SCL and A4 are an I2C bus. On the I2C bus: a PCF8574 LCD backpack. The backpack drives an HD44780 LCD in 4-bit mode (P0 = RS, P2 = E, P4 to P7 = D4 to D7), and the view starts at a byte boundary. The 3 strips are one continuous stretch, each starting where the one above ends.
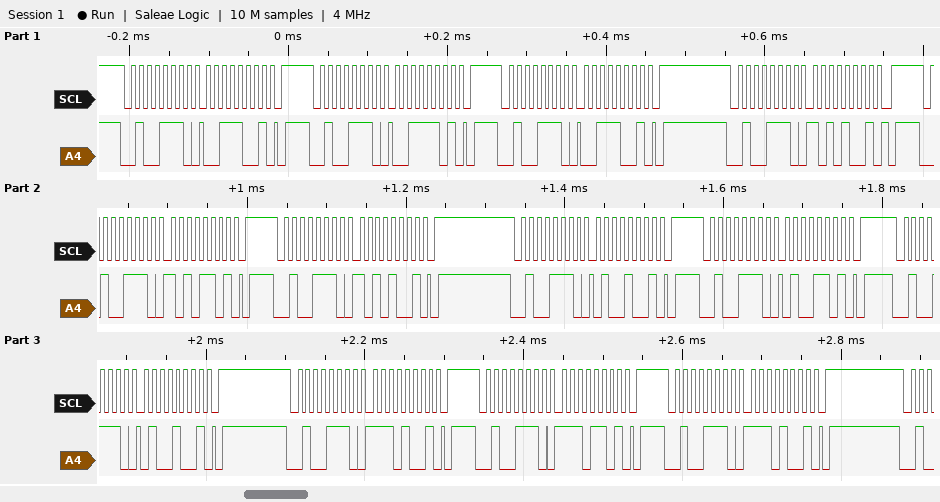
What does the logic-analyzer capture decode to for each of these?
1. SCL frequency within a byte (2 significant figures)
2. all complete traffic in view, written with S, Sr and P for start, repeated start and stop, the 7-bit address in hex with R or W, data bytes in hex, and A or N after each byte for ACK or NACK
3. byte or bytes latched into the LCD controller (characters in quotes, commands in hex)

100 kHz
S 27W A 39 A P S 27W A 3D A P S 27W A 39 A P S 27W A A9 A P S 27W A AD A P S 27W A A9 A P S 27W A 49 A P S 27W A 4D A P S 27W A 49 A P S 27W A E9 A P S 27W A ED A P S 27W A E9 A P
':' 'N'
